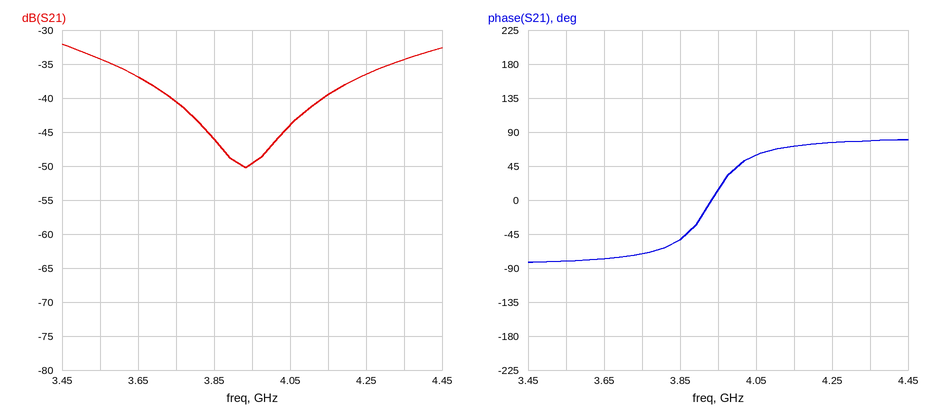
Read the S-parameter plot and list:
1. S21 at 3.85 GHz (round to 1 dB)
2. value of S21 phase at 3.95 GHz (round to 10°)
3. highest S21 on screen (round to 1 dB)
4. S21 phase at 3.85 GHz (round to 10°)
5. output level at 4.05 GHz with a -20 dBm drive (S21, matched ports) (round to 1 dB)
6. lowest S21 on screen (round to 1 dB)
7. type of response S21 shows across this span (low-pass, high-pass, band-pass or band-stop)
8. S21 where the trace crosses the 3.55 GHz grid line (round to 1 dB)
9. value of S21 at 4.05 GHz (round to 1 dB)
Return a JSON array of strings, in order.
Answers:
["-46 dB", "10°", "-32 dB", "-50°", "-64 dBm", "-50 dB", "band-stop", "-34 dB", "-44 dB"]
